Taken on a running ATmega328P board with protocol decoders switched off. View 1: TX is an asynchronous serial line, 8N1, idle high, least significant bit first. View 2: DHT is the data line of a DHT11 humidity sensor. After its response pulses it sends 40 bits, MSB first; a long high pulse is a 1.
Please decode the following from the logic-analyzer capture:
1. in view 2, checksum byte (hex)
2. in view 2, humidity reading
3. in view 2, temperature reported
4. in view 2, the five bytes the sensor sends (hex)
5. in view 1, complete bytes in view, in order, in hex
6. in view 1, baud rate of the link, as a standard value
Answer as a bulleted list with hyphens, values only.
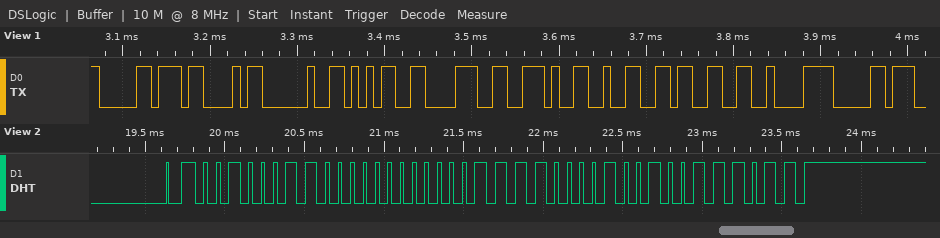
- 0x3B
- 35 %
- 15.9 °C
- 23 00 0F 09 3B
- B0 43 20 35 38 2E 32 33 C2 B0
- 115200 baud
